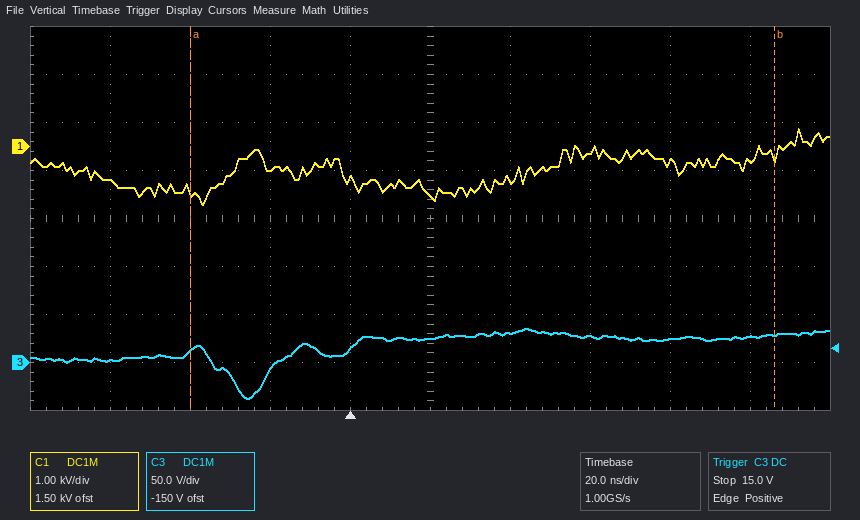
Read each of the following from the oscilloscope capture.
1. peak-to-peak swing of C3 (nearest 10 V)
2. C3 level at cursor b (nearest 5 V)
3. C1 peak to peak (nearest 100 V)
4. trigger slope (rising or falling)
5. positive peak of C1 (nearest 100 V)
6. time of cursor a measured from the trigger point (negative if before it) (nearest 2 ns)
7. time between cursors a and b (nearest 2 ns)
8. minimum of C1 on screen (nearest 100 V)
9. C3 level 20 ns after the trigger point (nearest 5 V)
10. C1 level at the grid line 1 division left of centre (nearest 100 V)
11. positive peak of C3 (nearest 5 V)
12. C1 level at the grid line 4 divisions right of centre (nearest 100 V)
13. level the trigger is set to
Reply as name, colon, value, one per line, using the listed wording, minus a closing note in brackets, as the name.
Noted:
peak-to-peak swing of C3: 70 V
C3 level at cursor b: 30 V
C1 peak to peak: 1.6 kV
trigger slope: rising
positive peak of C1: 400 V
time of cursor a measured from the trigger point (negative if before it): -40 ns
time between cursors a and b: 146 ns
minimum of C1 on screen: -1.2 kV
C3 level 20 ns after the trigger point: 25 V
C1 level at the grid line 1 division left of centre: -700 V
positive peak of C3: 35 V
C1 level at the grid line 4 divisions right of centre: -300 V
level the trigger is set to: 15.0 V
